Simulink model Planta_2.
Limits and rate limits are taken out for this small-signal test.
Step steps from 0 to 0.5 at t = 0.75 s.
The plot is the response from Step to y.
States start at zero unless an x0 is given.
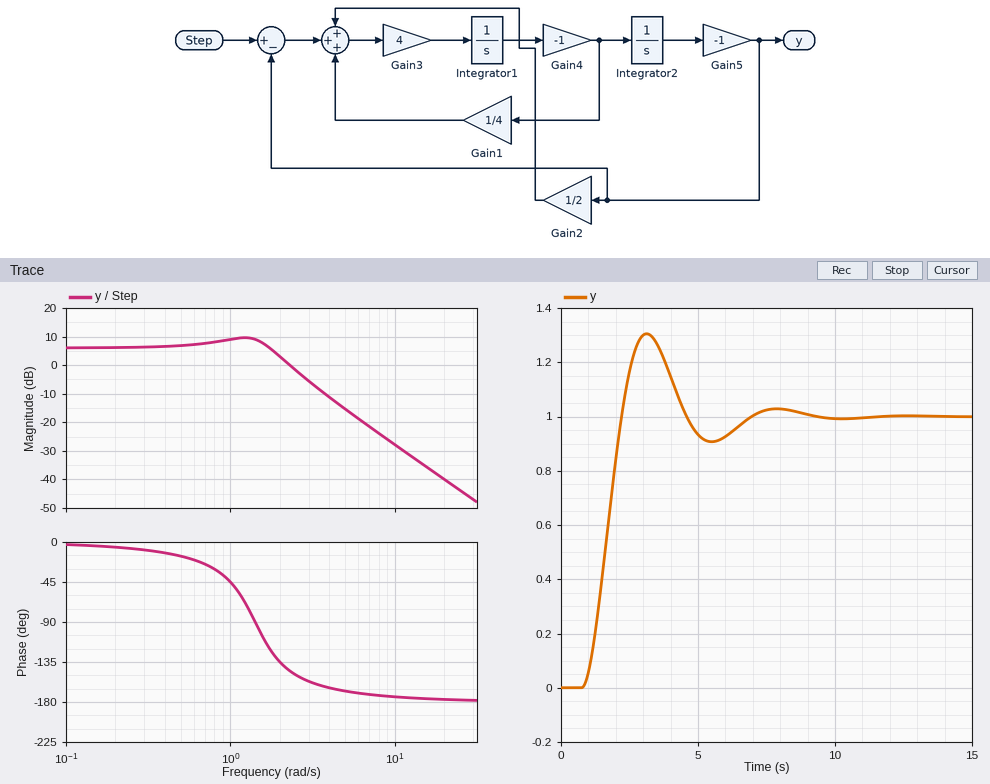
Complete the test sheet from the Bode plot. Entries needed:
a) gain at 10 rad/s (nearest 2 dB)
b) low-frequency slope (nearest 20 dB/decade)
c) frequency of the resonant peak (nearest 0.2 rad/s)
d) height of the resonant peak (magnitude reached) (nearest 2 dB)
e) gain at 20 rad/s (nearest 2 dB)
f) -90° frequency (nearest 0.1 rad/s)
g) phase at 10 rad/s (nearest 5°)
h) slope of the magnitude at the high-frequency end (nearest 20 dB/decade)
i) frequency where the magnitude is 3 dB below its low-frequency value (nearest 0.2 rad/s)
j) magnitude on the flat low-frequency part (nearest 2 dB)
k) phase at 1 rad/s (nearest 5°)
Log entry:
-28 dB
0 dB/decade
1.2 rad/s
10 dB
-40 dB
1.4 rad/s
-175°
-40 dB/decade
2.0 rad/s
6 dB
-45°
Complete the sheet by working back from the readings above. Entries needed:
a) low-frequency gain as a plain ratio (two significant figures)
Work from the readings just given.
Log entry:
2.0
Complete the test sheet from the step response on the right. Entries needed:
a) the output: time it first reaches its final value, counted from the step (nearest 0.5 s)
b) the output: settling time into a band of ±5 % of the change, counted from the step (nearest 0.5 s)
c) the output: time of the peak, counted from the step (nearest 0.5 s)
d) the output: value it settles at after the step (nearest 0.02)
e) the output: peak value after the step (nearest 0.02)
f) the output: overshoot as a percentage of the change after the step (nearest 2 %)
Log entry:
1.5 s
5.5 s
2.5 s
1.00
1.30
30 %
